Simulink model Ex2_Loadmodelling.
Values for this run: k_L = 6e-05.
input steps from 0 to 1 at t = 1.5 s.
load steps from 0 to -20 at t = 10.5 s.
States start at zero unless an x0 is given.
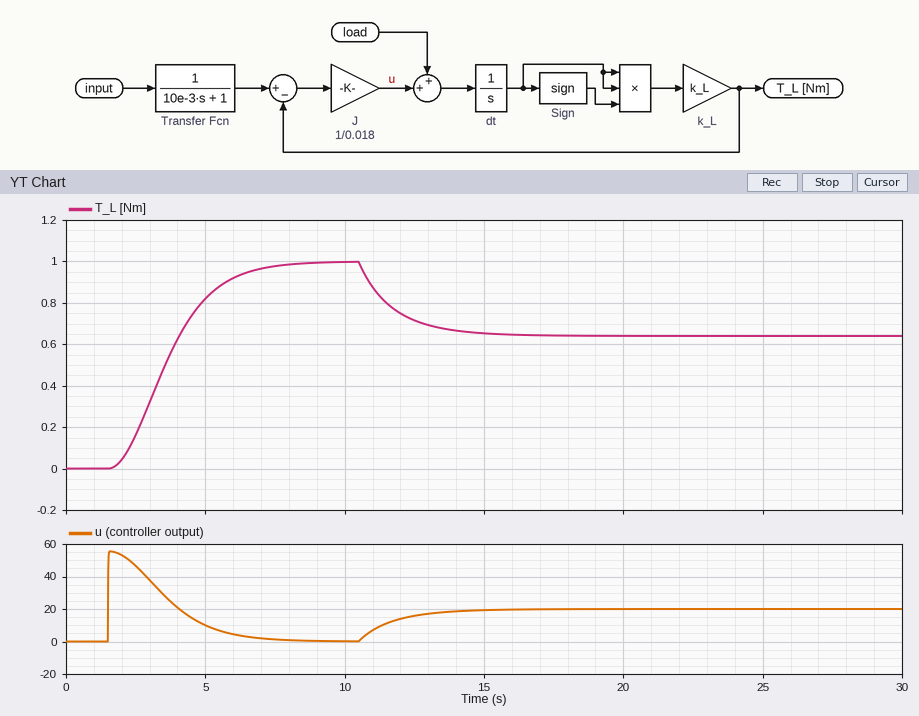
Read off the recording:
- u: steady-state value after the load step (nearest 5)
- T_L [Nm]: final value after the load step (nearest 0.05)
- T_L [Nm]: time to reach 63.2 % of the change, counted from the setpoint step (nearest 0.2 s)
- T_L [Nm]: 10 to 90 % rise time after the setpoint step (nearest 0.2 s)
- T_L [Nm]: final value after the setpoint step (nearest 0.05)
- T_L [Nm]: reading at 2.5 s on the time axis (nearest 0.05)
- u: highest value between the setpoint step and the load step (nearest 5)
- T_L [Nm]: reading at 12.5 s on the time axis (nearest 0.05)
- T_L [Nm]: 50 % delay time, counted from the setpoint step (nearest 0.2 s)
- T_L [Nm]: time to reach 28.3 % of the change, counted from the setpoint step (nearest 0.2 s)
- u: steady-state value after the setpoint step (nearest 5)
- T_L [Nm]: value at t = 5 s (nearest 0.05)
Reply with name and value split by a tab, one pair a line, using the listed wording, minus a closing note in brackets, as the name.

u: steady-state value after the load step	20
T_L [Nm]: final value after the load step	0.65
T_L [Nm]: time to reach 63.2 % of the change, counted from the setpoint step	2.6 s
T_L [Nm]: 10 to 90 % rise time after the setpoint step	3.4 s
T_L [Nm]: final value after the setpoint step	1.00
T_L [Nm]: reading at 2.5 s on the time axis	0.15
u: highest value between the setpoint step and the load step	55
T_L [Nm]: reading at 12.5 s on the time axis	0.70
T_L [Nm]: 50 % delay time, counted from the setpoint step	2.0 s
T_L [Nm]: time to reach 28.3 % of the change, counted from the setpoint step	1.4 s
u: steady-state value after the setpoint step	0
T_L [Nm]: value at t = 5 s	0.80
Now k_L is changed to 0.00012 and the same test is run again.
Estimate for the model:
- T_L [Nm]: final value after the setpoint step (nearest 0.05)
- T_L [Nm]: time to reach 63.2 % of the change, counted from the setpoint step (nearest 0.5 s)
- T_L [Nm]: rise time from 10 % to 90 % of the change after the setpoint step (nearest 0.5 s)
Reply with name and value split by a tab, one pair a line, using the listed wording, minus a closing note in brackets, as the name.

T_L [Nm]: final value after the setpoint step	1.00
T_L [Nm]: time to reach 63.2 % of the change, counted from the setpoint step	2.0 s
T_L [Nm]: rise time from 10 % to 90 % of the change after the setpoint step	2.5 s
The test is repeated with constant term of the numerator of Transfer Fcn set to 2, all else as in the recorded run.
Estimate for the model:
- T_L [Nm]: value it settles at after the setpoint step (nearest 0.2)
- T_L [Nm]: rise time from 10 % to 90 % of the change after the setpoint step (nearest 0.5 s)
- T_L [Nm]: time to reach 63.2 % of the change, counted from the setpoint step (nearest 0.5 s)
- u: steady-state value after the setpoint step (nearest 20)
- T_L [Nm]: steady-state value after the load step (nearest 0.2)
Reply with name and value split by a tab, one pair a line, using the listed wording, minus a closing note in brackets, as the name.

T_L [Nm]: value it settles at after the setpoint step	2.0
T_L [Nm]: rise time from 10 % to 90 % of the change after the setpoint step	2.5 s
T_L [Nm]: time to reach 63.2 % of the change, counted from the setpoint step	2.0 s
u: steady-state value after the setpoint step	0
T_L [Nm]: steady-state value after the load step	1.6
